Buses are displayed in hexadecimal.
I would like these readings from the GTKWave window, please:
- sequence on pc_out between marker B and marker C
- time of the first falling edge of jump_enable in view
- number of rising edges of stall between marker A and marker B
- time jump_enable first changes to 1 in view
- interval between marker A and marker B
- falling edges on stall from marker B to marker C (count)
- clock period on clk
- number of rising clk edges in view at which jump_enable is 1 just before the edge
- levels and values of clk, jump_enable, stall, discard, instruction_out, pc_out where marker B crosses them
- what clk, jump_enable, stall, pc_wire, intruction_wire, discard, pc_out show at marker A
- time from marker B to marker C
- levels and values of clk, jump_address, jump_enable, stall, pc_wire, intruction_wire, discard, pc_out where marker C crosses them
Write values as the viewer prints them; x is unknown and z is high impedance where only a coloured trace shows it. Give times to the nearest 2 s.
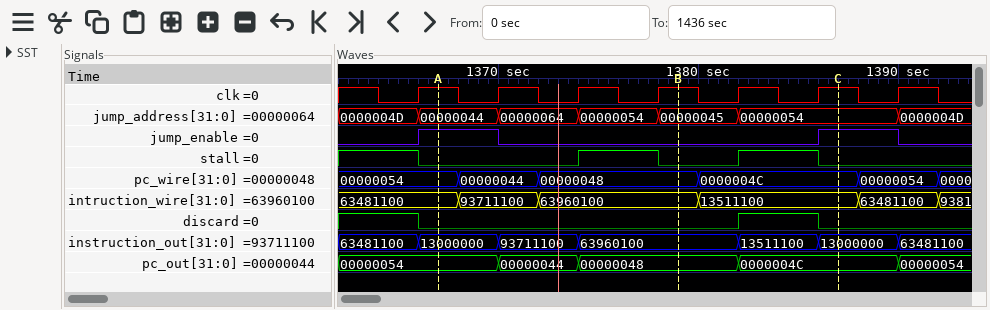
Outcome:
00000048, 0000004C
1370 s
1
1366 s
12 s
1
4 s
2
clk=1, jump_enable=0, stall=0, discard=0, instruction_out=63960100, pc_out=00000048
clk=1, jump_enable=1, stall=0, pc_wire=00000054, intruction_wire=63481100, discard=0, pc_out=00000054
8 s
clk=1, jump_address=00000054, jump_enable=1, stall=0, pc_wire=0000004C, intruction_wire=13511100, discard=0, pc_out=0000004C
